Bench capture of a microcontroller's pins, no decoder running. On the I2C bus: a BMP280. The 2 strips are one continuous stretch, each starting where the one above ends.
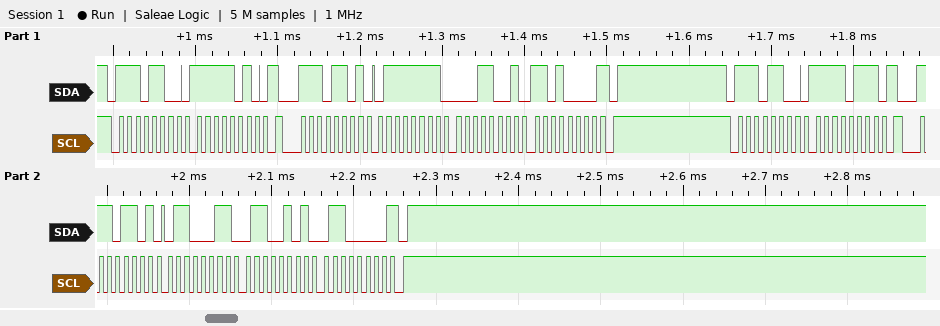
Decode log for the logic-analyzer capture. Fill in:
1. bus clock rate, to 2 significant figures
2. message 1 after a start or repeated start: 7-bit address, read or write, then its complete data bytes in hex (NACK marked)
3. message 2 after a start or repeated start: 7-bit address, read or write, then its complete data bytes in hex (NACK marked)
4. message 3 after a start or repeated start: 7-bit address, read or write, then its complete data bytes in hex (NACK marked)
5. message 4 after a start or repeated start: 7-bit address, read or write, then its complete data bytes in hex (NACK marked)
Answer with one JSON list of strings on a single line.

["100 kHz", "0x76 write: FA", "0x76 read: 7F 19 D0 NACK", "0x76 write: F7", "0x76 read: 63 65 60 NACK"]
